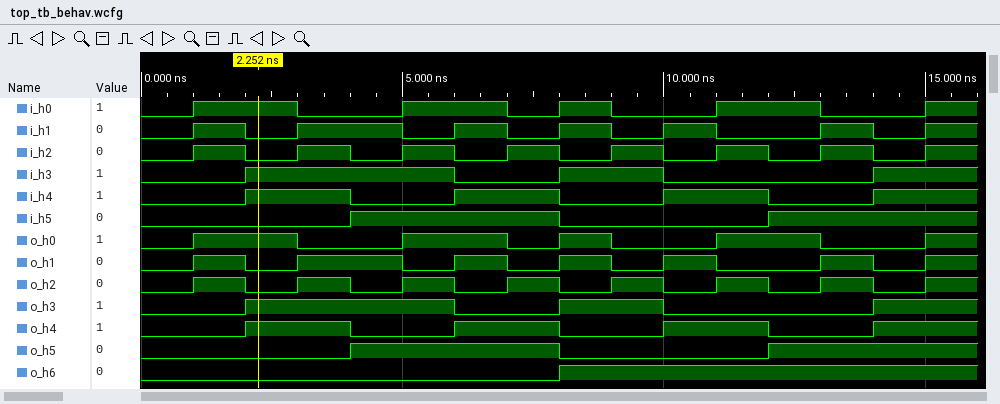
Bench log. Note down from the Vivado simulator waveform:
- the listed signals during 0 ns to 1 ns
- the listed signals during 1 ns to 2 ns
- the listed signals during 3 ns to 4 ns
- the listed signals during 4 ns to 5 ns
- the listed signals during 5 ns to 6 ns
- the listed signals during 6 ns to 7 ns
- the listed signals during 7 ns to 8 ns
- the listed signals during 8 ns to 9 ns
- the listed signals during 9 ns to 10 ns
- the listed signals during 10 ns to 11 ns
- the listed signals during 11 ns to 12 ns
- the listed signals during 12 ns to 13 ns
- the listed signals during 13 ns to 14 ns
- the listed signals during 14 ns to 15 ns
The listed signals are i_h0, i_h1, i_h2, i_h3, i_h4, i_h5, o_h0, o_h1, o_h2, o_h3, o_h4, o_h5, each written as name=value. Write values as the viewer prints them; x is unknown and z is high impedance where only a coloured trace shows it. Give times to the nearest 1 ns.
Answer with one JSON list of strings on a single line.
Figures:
["i_h0=0, i_h1=0, i_h2=0, i_h3=0, i_h4=0, i_h5=0, o_h0=0, o_h1=0, o_h2=0, o_h3=0, o_h4=0, o_h5=0", "i_h0=1, i_h1=1, i_h2=1, i_h3=0, i_h4=0, i_h5=0, o_h0=1, o_h1=1, o_h2=1, o_h3=0, o_h4=0, o_h5=0", "i_h0=0, i_h1=1, i_h2=1, i_h3=1, i_h4=1, i_h5=0, o_h0=0, o_h1=1, o_h2=1, o_h3=1, o_h4=1, o_h5=0", "i_h0=0, i_h1=1, i_h2=0, i_h3=1, i_h4=0, i_h5=1, o_h0=0, o_h1=1, o_h2=0, o_h3=1, o_h4=0, o_h5=1", "i_h0=1, i_h1=0, i_h2=1, i_h3=1, i_h4=0, i_h5=1, o_h0=1, o_h1=0, o_h2=1, o_h3=1, o_h4=0, o_h5=1", "i_h0=1, i_h1=1, i_h2=0, i_h3=0, i_h4=1, i_h5=1, o_h0=1, o_h1=1, o_h2=0, o_h3=0, o_h4=1, o_h5=1", "i_h0=0, i_h1=0, i_h2=1, i_h3=0, i_h4=1, i_h5=1, o_h0=0, o_h1=0, o_h2=1, o_h3=0, o_h4=1, o_h5=1", "i_h0=1, i_h1=1, i_h2=0, i_h3=1, i_h4=0, i_h5=0, o_h0=1, o_h1=1, o_h2=0, o_h3=1, o_h4=0, o_h5=0", "i_h0=0, i_h1=0, i_h2=1, i_h3=1, i_h4=0, i_h5=0, o_h0=0, o_h1=0, o_h2=1, o_h3=1, o_h4=0, o_h5=0", "i_h0=0, i_h1=1, i_h2=0, i_h3=0, i_h4=1, i_h5=0, o_h0=0, o_h1=1, o_h2=0, o_h3=0, o_h4=1, o_h5=0", "i_h0=1, i_h1=0, i_h2=1, i_h3=0, i_h4=1, i_h5=0, o_h0=1, o_h1=0, o_h2=1, o_h3=0, o_h4=1, o_h5=0", "i_h0=1, i_h1=0, i_h2=0, i_h3=0, i_h4=0, i_h5=1, o_h0=1, o_h1=0, o_h2=0, o_h3=0, o_h4=0, o_h5=1", "i_h0=0, i_h1=1, i_h2=1, i_h3=0, i_h4=0, i_h5=1, o_h0=0, o_h1=1, o_h2=1, o_h3=0, o_h4=0, o_h5=1", "i_h0=0, i_h1=0, i_h2=0, i_h3=1, i_h4=1, i_h5=1, o_h0=0, o_h1=0, o_h2=0, o_h3=1, o_h4=1, o_h5=1"]
